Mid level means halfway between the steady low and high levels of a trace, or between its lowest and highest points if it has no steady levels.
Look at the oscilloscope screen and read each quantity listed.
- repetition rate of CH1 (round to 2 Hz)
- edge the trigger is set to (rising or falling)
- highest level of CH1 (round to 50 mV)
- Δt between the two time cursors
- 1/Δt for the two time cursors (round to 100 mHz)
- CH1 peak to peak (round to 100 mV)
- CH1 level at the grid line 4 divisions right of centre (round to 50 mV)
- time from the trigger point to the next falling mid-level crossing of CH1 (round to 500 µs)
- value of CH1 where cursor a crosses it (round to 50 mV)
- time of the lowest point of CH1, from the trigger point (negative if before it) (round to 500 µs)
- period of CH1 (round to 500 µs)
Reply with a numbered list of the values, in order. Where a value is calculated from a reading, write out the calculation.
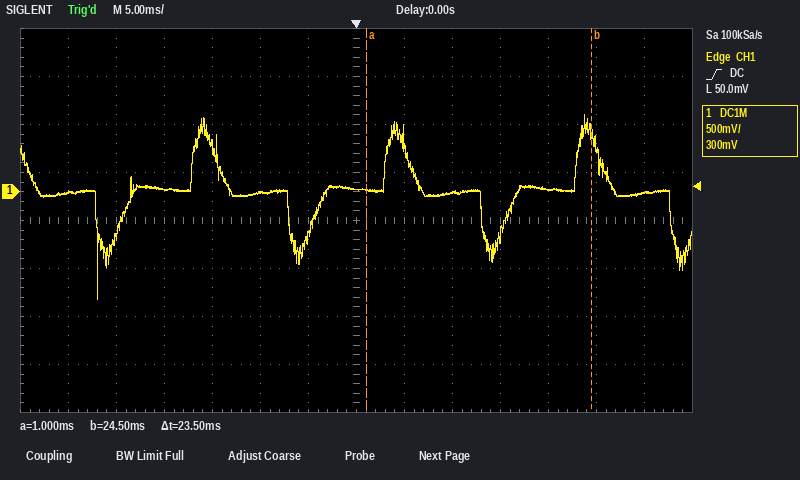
1. 1 / 20.0 ms ≈ 50 Hz
2. rising
3. 800 mV
4. 23.5 ms
5. 1 / 23.5 ms ≈ 42.6 Hz
6. 1.90 V
7. 0 mV
8. 13.0 ms
9. 0 mV
10. -27.0 ms
11. 20.0 ms
